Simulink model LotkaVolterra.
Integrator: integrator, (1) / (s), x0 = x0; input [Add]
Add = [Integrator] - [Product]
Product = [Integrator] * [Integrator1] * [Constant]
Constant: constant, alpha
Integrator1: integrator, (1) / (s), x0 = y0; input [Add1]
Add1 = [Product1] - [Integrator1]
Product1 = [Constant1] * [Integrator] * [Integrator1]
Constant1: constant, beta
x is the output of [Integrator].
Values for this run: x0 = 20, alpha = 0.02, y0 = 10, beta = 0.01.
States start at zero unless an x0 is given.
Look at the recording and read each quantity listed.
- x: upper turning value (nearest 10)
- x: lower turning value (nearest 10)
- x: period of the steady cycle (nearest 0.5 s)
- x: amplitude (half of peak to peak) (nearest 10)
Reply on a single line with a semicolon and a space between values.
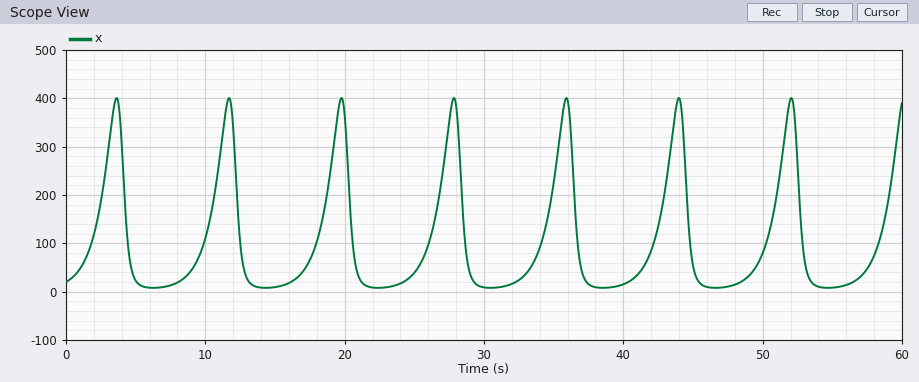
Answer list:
400; 10; 8.0 s; 200
